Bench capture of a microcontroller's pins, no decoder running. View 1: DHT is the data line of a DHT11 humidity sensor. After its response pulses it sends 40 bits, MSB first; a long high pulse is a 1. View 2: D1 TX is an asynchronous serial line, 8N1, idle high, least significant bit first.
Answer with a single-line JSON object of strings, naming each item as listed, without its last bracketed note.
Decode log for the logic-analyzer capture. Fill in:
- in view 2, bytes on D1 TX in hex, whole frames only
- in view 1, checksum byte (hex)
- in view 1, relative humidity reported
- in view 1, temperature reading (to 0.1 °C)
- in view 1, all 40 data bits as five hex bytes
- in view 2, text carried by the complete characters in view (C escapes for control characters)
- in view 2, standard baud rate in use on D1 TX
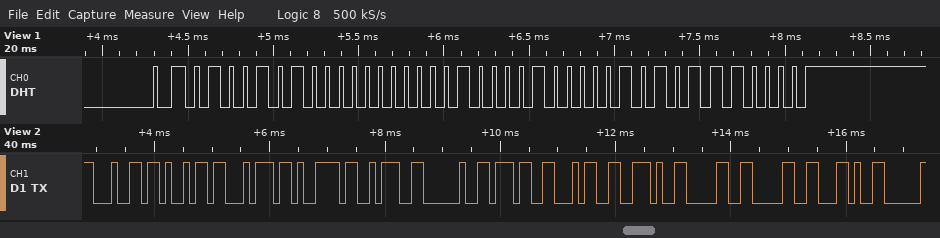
{"in view 2, bytes on D1 TX in hex, whole frames only": "64 69 74 79 3A 20 37 34 2E 30 30 2C", "in view 1, checksum byte": "0x70", "in view 1, relative humidity reported": "74 %", "in view 1, temperature reading": "33.5 °C", "in view 1, all 40 data bits as five hex bytes": "4A 00 21 05 70", "in view 2, text carried by the complete characters in view": "\"dity: 74.00,\"", "in view 2, standard baud rate in use on D1 TX": "9600 baud"}
